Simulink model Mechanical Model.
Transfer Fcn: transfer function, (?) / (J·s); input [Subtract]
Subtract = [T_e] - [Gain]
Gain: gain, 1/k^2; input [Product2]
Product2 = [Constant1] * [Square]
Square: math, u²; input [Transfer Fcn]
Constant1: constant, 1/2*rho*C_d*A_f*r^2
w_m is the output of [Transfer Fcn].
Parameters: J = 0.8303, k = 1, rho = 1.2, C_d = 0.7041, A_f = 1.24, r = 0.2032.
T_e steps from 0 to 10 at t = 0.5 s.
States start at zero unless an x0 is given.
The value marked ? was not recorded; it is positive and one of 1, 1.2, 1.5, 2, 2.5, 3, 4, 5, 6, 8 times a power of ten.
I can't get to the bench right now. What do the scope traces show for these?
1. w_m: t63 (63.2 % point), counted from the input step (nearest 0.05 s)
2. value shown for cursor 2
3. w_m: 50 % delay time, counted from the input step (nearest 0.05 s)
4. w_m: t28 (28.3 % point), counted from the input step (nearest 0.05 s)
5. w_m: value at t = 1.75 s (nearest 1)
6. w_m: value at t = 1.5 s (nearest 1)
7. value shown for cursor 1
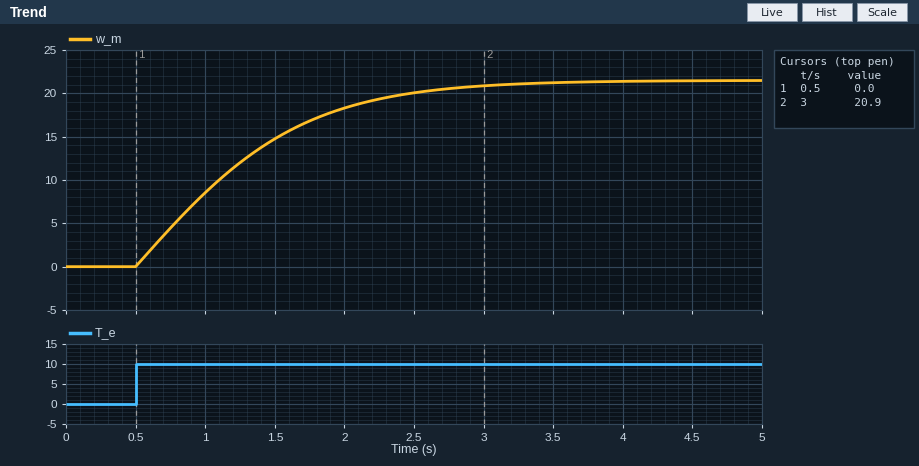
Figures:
0.90 s
20.9
0.65 s
0.35 s
17
15
0.0
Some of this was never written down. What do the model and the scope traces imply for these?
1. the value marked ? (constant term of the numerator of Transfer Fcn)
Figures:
1.5
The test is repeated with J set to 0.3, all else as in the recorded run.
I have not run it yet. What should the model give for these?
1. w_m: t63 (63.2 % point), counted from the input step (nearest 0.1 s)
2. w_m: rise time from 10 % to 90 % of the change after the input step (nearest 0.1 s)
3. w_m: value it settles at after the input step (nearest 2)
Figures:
0.3 s
0.6 s
22
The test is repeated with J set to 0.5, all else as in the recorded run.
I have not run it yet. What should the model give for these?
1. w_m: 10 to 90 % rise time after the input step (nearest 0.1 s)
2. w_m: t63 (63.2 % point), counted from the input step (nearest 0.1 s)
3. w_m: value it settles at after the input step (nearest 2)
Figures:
1.0 s
0.5 s
22
